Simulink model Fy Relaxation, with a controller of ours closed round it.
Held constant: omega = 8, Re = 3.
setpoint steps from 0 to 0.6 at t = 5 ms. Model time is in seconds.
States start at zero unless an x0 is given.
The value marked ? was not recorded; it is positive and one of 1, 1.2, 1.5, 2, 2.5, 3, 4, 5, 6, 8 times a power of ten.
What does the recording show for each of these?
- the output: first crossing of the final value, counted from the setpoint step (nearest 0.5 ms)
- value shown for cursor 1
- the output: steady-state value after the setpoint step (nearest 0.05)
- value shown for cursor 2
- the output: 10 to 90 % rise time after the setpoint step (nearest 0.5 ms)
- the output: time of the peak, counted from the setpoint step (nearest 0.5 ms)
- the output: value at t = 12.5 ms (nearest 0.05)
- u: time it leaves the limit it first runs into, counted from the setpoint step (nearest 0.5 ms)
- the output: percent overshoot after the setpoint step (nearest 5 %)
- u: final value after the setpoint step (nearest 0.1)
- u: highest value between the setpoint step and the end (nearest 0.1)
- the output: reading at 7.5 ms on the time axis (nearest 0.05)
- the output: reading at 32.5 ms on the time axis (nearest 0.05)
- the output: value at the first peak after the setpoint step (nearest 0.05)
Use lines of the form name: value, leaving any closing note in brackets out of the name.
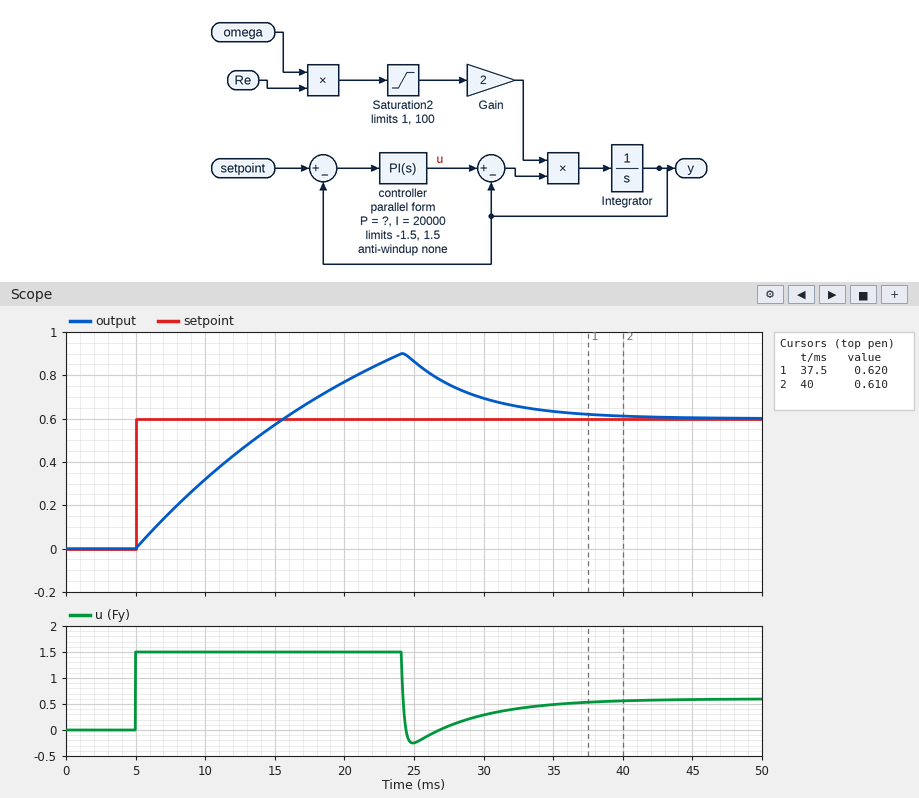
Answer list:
the output: first crossing of the final value, counted from the setpoint step: 10.5 ms
value shown for cursor 1: 0.620
the output: steady-state value after the setpoint step: 0.60
value shown for cursor 2: 0.610
the output: 10 to 90 % rise time after the setpoint step: 8.5 ms
the output: time of the peak, counted from the setpoint step: 19.0 ms
the output: value at t = 12.5 ms: 0.45
u: time it leaves the limit it first runs into, counted from the setpoint step: 19.0 ms
the output: percent overshoot after the setpoint step: 50 %
u: final value after the setpoint step: 0.6
u: highest value between the setpoint step and the end: 1.5
the output: reading at 7.5 ms on the time axis: 0.15
the output: reading at 32.5 ms on the time axis: 0.65
the output: value at the first peak after the setpoint step: 0.90
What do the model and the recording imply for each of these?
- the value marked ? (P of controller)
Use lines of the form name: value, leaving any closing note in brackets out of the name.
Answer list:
the value marked ?: 100
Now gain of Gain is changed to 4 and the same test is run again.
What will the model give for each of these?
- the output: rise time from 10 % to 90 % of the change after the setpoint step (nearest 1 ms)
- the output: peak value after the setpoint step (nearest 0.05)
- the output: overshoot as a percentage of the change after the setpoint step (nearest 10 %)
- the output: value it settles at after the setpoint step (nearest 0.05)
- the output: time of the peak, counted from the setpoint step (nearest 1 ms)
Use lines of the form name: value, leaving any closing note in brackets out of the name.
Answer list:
the output: rise time from 10 % to 90 % of the change after the setpoint step: 4 ms
the output: peak value after the setpoint step: 0.80
the output: overshoot as a percentage of the change after the setpoint step: 40 %
the output: value it settles at after the setpoint step: 0.60
the output: time of the peak, counted from the setpoint step: 8 ms
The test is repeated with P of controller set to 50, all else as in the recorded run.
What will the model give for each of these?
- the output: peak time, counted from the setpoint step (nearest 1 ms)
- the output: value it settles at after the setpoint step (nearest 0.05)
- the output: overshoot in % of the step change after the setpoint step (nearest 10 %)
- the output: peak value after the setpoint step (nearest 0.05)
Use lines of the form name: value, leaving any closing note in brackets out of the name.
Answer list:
the output: peak time, counted from the setpoint step: 21 ms
the output: value it settles at after the setpoint step: 0.60
the output: overshoot in % of the step change after the setpoint step: 60 %
the output: peak value after the setpoint step: 0.95
